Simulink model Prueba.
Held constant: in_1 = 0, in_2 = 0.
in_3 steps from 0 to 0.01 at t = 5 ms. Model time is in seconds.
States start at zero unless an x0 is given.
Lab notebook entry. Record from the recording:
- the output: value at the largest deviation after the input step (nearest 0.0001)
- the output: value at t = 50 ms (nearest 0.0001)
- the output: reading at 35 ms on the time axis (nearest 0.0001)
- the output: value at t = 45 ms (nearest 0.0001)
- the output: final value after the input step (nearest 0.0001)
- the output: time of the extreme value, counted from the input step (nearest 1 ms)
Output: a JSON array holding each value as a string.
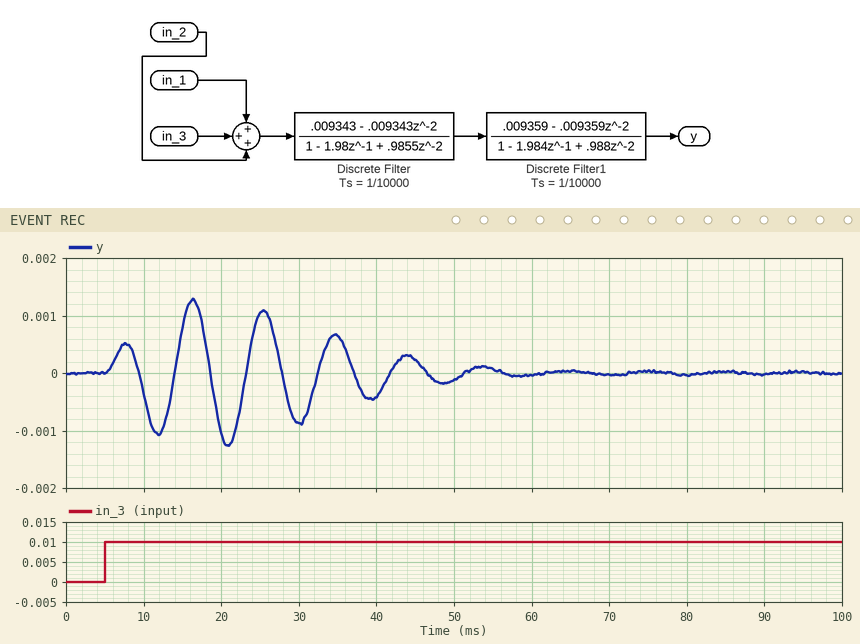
["0.0013", "-0.0001", "0.0006", "0.0002", "0.0000", "11 ms"]
